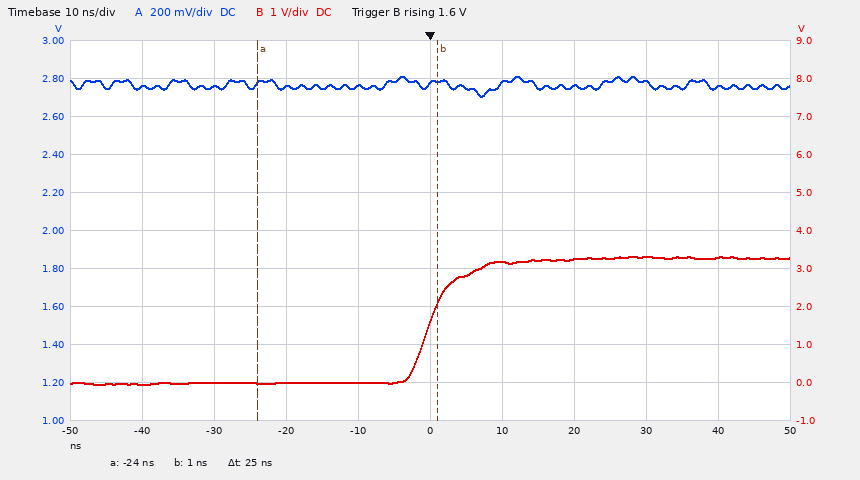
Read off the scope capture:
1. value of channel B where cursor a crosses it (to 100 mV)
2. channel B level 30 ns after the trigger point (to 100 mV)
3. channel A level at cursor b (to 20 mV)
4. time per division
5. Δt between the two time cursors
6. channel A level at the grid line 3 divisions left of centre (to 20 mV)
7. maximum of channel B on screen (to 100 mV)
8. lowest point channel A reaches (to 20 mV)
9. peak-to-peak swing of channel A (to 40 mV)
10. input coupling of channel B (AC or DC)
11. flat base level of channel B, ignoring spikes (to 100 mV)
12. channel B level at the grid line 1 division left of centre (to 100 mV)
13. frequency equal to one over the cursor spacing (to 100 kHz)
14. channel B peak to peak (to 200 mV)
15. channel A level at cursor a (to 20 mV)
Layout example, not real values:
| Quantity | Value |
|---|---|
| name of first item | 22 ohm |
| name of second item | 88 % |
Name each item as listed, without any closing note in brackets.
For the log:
| Quantity | Value |
|---|---|
| value of channel B where cursor a crosses it | 0.0 V |
| channel B level 30 ns after the trigger point | 3.3 V |
| channel A level at cursor b | 2.78 V |
| time per division | 10 ns |
| Δt between the two time cursors | 25 ns |
| channel A level at the grid line 3 divisions left of centre | 2.76 V |
| maximum of channel B on screen | 3.3 V |
| lowest point channel A reaches | 2.70 V |
| peak-to-peak swing of channel A | 120 mV |
| input coupling of channel B | DC |
| flat base level of channel B, ignoring spikes | 0.0 V |
| channel B level at the grid line 1 division left of centre | 0.0 V |
| frequency equal to one over the cursor spacing | 40.0 MHz |
| channel B peak to peak | 3.4 V |
| channel A level at cursor a | 2.78 V |
